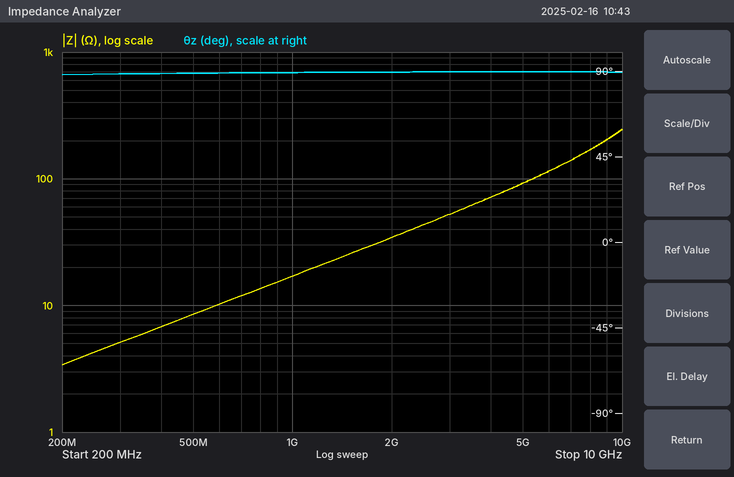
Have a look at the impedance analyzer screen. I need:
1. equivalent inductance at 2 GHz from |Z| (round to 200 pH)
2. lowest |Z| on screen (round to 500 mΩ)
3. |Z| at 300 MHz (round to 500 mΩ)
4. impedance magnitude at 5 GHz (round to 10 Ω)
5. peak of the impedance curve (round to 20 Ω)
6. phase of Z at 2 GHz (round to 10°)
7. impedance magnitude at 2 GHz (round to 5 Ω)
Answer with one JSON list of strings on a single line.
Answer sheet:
["2.8 nH", "3.5 Ω", "5.0 Ω", "90 Ω", "240 Ω", "90°", "35 Ω"]
